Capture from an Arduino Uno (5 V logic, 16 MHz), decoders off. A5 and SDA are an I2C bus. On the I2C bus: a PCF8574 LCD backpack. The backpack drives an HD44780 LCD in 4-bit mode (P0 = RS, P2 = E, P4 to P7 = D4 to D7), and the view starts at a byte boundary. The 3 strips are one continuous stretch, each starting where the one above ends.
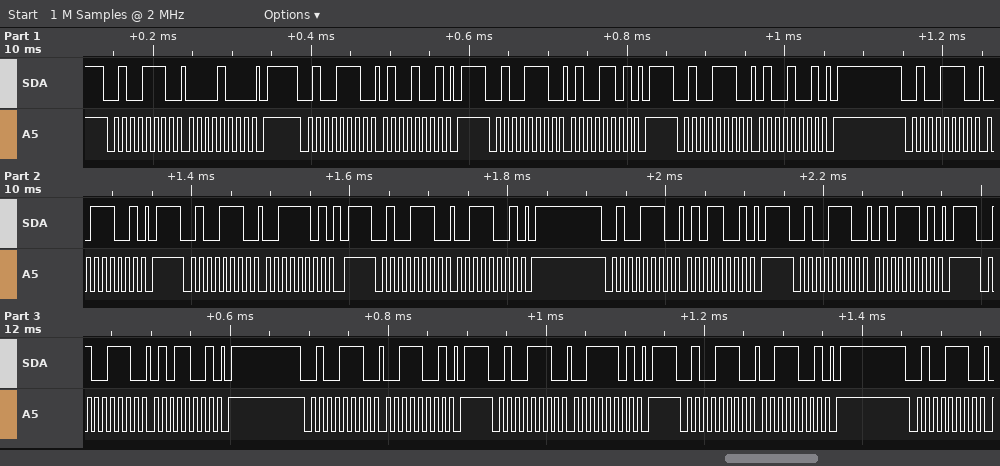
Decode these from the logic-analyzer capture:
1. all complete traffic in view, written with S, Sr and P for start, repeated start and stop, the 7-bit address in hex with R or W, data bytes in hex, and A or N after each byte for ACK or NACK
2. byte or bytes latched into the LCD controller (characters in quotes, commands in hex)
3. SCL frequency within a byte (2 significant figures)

S 27W A 08 A P S 27W A 49 A P S 27W A 4D A P S 27W A 49 A P S 27W A 39 A P S 27W A 3D A P S 27W A 39 A P S 27W A 59 A P S 27W A 5D A P S 27W A 59 A P S 27W A 39 A P S 27W A 3D A P S 27W A 39 A P S 27W A
'C' 'S'
100 kHz
